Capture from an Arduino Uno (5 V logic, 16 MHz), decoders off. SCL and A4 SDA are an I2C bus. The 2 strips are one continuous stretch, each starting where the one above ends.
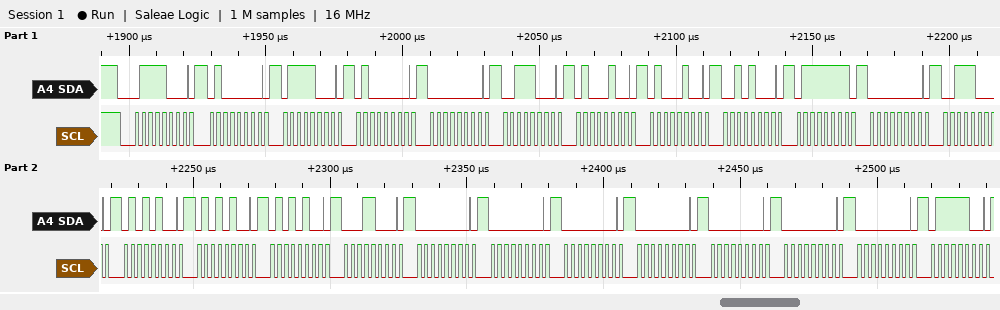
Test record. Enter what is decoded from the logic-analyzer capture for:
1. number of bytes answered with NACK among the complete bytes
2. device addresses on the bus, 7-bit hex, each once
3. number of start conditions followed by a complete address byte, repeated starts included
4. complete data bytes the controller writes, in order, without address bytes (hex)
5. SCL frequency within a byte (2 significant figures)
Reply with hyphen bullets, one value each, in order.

- 0
- 0x3C
- 1
- 40 78 40 00 38 44 44 28 7F 00 38 54 54 54 18 00 00 00 00 00 00 00 7C
- 400 kHz
